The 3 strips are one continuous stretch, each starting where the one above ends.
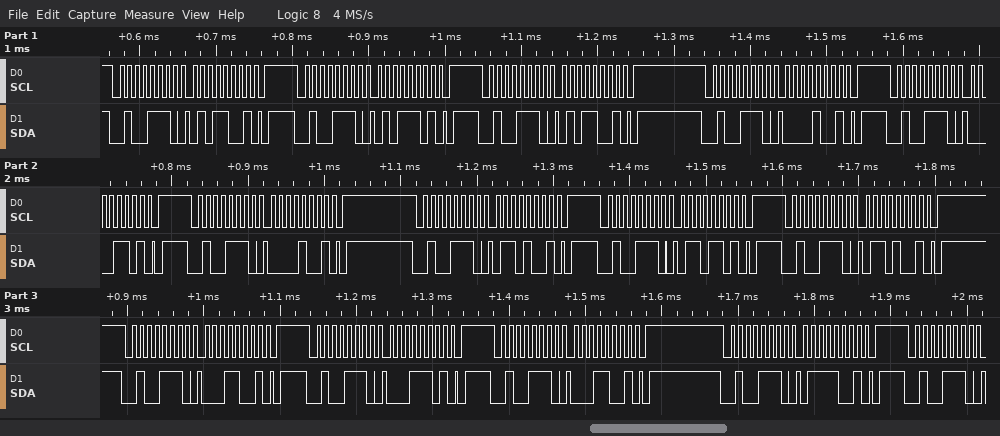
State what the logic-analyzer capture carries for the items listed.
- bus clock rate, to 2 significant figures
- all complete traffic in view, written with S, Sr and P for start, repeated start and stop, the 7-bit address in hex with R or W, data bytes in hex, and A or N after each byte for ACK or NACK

100 kHz
S 27W A 59 A P S 27W A 5D A P S 27W A 59 A P S 27W A 09 A P S 27W A 0D A P S 27W A 09 A P S 27W A 69 A P S 27W A 6D A P S 27W A 69 A P S 27W A 19 A P S 27W A 1D A P S 27W A 19 A P S 27W A 79 A P S 27W A
